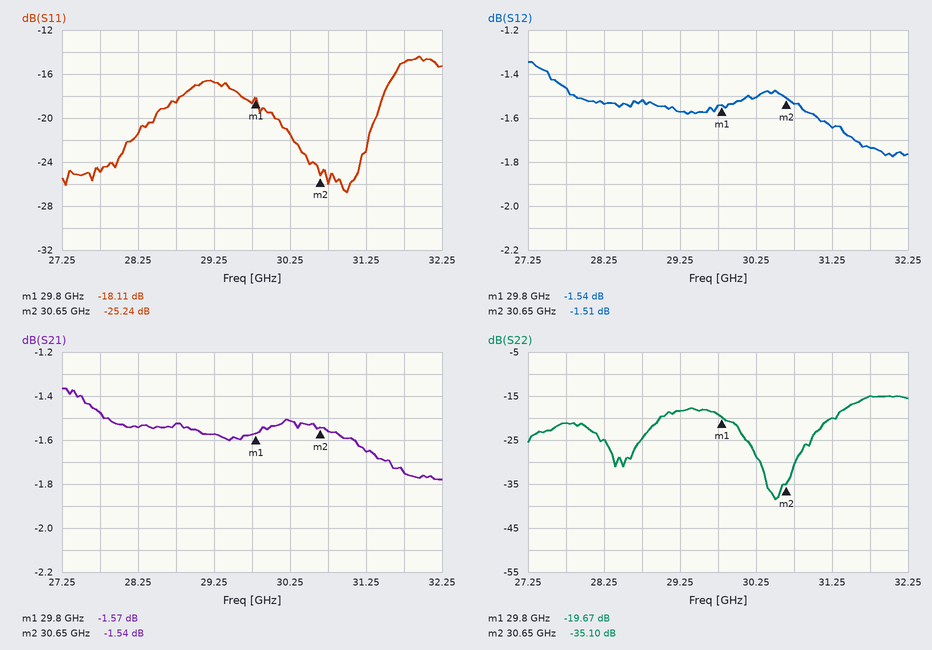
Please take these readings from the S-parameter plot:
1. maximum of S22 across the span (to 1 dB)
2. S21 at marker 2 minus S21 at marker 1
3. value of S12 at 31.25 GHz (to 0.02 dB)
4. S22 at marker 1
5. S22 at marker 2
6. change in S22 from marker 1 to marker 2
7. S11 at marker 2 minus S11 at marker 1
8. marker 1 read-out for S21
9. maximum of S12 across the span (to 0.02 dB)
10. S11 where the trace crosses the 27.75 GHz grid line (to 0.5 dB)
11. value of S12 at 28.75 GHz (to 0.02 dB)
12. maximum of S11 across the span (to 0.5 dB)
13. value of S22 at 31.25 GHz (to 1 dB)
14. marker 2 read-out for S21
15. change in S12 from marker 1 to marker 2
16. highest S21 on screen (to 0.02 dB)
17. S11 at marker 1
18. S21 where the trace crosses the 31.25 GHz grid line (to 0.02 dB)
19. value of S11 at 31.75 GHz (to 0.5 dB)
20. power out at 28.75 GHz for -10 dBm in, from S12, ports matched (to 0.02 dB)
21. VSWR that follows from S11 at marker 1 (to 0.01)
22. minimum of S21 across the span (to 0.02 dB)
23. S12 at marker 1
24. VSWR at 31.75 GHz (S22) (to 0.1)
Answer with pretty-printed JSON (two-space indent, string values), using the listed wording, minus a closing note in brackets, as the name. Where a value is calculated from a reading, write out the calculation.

{
  "maximum of S22 across the span": "-15 dB",
  "S21 at marker 2 minus S21 at marker 1": "-1.54 − (-1.57) = 0.03 dB",
  "value of S12 at 31.25 GHz": "-1.64 dB",
  "S22 at marker 1": "-19.67 dB",
  "S22 at marker 2": "-35.10 dB",
  "change in S22 from marker 1 to marker 2": "-35.1 − (-19.67) = -15.43 dB",
  "S11 at marker 2 minus S11 at marker 1": "-25.24 − (-18.11) = -7.13 dB",
  "marker 1 read-out for S21": "-1.57 dB",
  "maximum of S12 across the span": "-1.34 dB",
  "S11 where the trace crosses the 27.75 GHz grid line": "-25.0 dB",
  "value of S12 at 28.75 GHz": "-1.52 dB",
  "maximum of S11 across the span": "-14.5 dB",
  "value of S22 at 31.25 GHz": "-20 dB",
  "marker 2 read-out for S21": "-1.54 dB",
  "change in S12 from marker 1 to marker 2": "-1.51 − (-1.54) = 0.03 dB",
  "highest S21 on screen": "-1.36 dB",
  "S11 at marker 1": "-18.11 dB",
  "S21 where the trace crosses the 31.25 GHz grid line": "-1.66 dB",
  "value of S11 at 31.75 GHz": "-15.0 dB",
  "power out at 28.75 GHz for -10 dBm in, from S12, ports matched": "-10 dBm + (-1.52 dB) = -11.52 dBm",
  "VSWR that follows from S11 at marker 1": "(1 + 0.1243)/(1 − 0.1243) ≈ 1.28",
  "minimum of S21 across the span": "-1.78 dB",
  "S12 at marker 1": "-1.54 dB",
  "VSWR at 31.75 GHz (S22)": "|Γ| = 10^(-15/20) = 0.1778; VSWR = (1 + 0.1778)/(1 − 0.1778) ≈ 1.4"
}
